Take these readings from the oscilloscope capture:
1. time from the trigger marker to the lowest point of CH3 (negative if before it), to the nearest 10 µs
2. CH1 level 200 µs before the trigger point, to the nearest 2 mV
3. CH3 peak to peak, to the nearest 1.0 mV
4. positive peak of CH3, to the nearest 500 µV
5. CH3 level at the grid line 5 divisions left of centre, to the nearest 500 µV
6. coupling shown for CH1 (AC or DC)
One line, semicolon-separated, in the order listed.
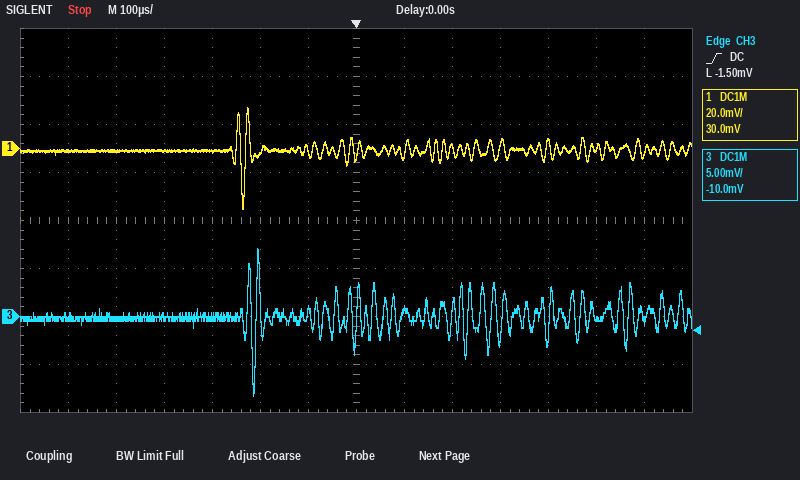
-210 µs; -2 mV; 15.0 mV; 7.0 mV; 0.0 mV; DC
